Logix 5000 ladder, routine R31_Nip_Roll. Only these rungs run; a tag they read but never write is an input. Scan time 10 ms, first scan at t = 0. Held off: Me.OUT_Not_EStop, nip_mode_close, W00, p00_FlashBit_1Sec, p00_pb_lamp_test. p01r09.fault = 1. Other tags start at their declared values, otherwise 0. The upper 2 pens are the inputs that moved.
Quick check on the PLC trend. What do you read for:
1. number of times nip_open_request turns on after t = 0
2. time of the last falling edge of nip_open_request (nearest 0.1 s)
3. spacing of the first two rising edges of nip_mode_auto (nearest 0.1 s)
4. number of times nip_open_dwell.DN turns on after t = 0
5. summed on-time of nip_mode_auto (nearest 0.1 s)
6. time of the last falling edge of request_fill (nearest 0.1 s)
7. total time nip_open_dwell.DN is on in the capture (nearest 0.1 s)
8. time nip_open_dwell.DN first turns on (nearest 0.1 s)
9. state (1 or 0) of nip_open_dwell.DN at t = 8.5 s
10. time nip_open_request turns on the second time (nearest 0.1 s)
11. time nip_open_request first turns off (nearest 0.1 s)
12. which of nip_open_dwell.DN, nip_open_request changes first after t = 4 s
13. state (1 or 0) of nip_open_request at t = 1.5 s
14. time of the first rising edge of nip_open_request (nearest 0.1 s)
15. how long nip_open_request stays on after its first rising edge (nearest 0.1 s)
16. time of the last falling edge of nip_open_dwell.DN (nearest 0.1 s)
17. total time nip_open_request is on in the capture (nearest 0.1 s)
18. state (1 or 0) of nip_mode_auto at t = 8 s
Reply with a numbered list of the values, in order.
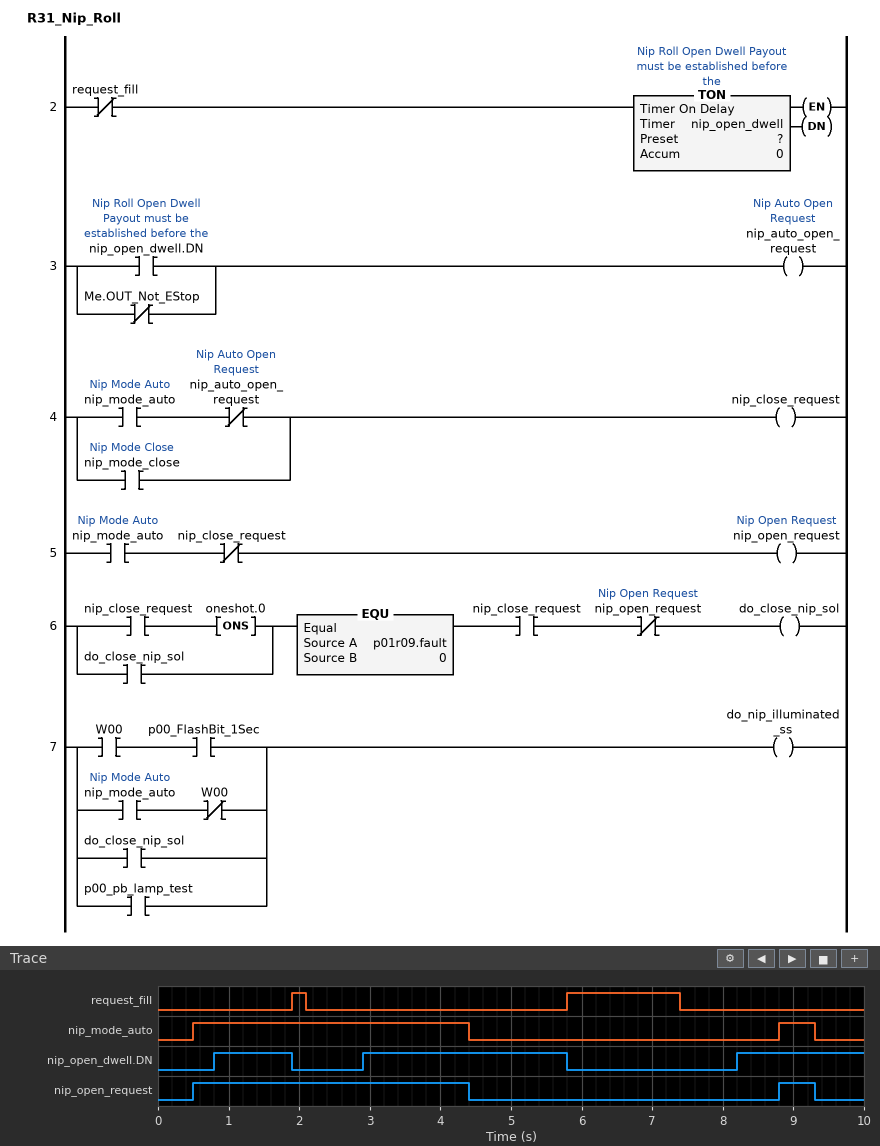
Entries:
1. 2
2. 9.3 s
3. 8.3 s
4. 3
5. 4.4 s
6. 7.4 s
7. 5.8 s
8. 0.8 s
9. 1
10. 8.8 s
11. 4.4 s
12. nip_open_request
13. 1
14. 0.5 s
15. 3.9 s
16. 5.8 s
17. 4.4 s
18. 0
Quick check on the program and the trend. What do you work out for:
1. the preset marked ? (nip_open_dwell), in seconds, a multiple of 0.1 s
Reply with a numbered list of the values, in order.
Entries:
1. 0.8 s
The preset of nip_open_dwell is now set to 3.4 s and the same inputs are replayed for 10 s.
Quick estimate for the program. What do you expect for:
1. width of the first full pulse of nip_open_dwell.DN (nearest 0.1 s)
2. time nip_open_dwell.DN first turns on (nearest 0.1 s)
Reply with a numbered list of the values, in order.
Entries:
1. 0.3 s
2. 5.5 s
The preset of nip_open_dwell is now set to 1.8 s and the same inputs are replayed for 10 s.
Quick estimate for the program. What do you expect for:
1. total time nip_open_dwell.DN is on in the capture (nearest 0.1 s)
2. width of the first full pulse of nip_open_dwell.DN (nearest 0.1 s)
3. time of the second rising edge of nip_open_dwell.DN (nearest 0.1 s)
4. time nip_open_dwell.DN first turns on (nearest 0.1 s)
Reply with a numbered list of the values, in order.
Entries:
1. 2.8 s
2. 0.1 s
3. 3.9 s
4. 1.8 s
